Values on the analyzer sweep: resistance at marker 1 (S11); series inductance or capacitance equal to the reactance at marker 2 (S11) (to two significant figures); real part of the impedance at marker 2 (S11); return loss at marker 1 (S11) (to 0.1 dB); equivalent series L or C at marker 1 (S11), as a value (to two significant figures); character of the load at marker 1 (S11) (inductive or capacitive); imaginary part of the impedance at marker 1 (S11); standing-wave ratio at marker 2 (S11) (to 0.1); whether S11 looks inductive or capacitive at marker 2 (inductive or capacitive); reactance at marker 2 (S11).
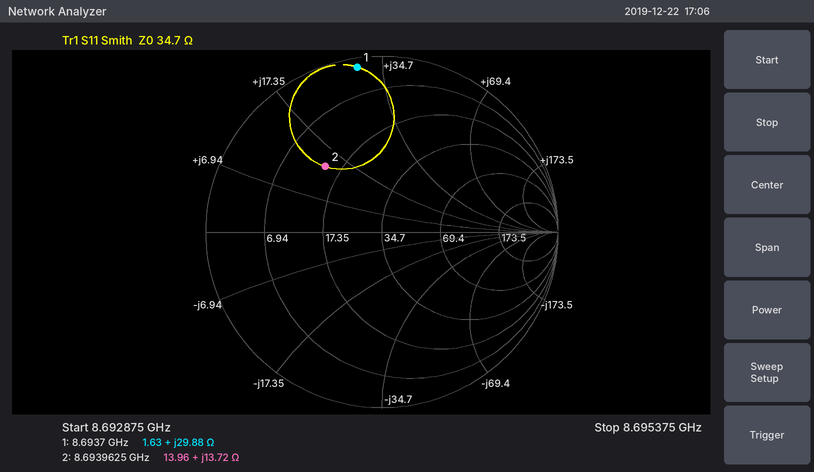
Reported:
1.63 Ω
250 pH
13.96 Ω
0.5 dB
550 pH
inductive
+29.88 Ω
2.9
inductive
+13.72 Ω
